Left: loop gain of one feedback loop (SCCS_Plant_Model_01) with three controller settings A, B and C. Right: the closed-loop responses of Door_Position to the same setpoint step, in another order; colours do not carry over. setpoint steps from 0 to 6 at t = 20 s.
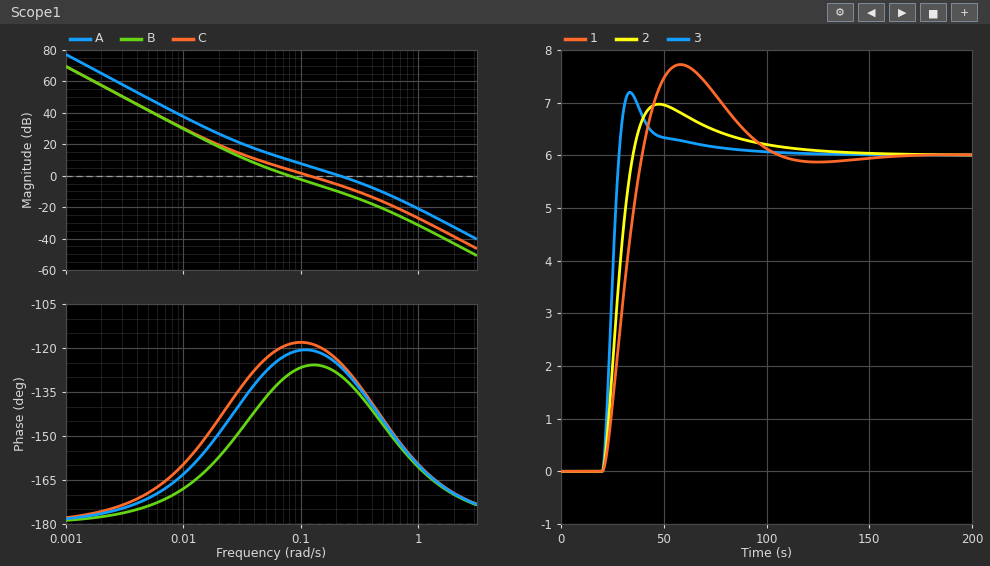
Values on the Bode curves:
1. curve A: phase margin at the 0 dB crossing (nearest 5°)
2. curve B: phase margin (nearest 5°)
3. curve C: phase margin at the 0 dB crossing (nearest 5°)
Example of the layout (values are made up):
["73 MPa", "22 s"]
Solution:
["55°", "50°", "60°"]
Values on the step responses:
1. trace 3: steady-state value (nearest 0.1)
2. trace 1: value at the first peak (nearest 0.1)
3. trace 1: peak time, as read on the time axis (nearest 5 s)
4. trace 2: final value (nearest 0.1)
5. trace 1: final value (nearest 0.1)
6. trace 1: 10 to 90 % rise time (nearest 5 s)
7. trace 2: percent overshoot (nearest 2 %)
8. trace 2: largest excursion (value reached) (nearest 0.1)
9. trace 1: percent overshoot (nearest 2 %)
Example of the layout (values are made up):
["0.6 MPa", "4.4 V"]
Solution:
["6.0", "7.7", "60 s", "6.0", "6.0", "15 s", "16 %", "7.0", "28 %"]
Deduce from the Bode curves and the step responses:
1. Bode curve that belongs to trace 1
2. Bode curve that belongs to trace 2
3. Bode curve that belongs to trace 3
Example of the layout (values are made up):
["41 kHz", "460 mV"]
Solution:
["B", "C", "A"]
